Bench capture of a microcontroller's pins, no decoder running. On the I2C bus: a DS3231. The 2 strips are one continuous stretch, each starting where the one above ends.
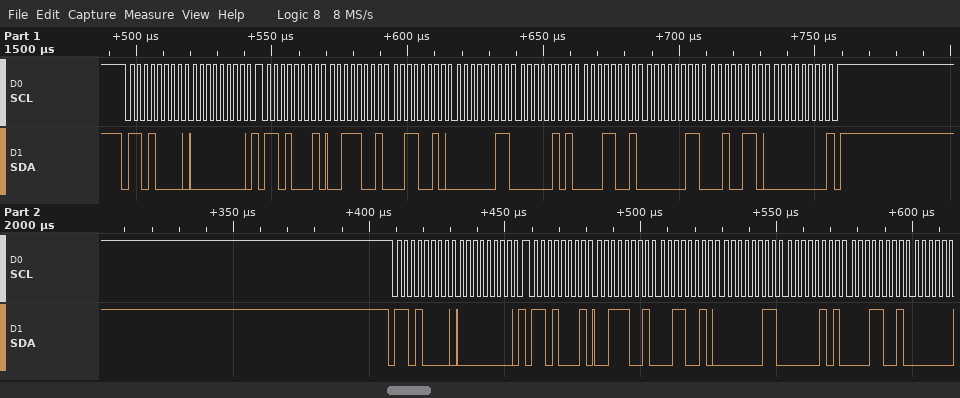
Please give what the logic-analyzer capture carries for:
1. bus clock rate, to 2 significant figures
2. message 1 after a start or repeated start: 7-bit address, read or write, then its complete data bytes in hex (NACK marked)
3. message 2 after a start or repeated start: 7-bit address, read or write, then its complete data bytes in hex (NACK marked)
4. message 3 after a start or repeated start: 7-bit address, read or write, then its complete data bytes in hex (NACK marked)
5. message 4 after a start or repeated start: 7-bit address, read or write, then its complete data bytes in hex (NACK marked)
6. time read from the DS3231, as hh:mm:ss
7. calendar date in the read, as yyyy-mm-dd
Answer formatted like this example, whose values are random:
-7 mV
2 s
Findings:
400 kHz
0x68 write: 00
0x68 read: 39 32 03 05 19 03 26 00 NACK
0x68 write: 00
0x68 read: 39 32 03 05 19
03:32:39
2026-03-19
